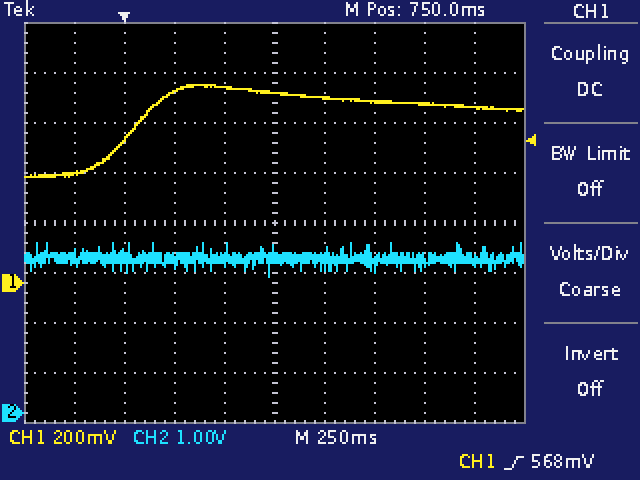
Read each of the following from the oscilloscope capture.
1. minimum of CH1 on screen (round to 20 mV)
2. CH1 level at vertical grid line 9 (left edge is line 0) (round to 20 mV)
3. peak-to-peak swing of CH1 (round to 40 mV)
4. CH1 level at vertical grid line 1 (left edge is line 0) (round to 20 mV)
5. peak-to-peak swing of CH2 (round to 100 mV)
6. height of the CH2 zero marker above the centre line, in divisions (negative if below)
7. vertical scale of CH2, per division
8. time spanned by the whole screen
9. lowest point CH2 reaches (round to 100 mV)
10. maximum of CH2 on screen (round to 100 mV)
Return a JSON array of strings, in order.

["420 mV", "700 mV", "360 mV", "440 mV", "700 mV", "-3.8 div", "1 V", "2.5 s", "2.7 V", "3.4 V"]
